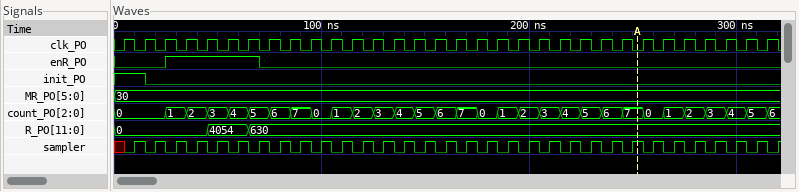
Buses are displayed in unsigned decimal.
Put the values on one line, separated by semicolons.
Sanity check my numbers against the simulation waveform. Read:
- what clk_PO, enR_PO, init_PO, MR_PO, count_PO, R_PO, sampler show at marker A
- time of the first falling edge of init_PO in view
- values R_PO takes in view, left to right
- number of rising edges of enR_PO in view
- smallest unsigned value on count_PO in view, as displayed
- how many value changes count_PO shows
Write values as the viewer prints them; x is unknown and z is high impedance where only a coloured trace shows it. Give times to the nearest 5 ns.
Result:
clk_PO=0, enR_PO=0, init_PO=0, MR_PO=30, count_PO=7, R_PO=630, sampler=1; 15 ns; 0, 4054, 630; 1; 0; 30
